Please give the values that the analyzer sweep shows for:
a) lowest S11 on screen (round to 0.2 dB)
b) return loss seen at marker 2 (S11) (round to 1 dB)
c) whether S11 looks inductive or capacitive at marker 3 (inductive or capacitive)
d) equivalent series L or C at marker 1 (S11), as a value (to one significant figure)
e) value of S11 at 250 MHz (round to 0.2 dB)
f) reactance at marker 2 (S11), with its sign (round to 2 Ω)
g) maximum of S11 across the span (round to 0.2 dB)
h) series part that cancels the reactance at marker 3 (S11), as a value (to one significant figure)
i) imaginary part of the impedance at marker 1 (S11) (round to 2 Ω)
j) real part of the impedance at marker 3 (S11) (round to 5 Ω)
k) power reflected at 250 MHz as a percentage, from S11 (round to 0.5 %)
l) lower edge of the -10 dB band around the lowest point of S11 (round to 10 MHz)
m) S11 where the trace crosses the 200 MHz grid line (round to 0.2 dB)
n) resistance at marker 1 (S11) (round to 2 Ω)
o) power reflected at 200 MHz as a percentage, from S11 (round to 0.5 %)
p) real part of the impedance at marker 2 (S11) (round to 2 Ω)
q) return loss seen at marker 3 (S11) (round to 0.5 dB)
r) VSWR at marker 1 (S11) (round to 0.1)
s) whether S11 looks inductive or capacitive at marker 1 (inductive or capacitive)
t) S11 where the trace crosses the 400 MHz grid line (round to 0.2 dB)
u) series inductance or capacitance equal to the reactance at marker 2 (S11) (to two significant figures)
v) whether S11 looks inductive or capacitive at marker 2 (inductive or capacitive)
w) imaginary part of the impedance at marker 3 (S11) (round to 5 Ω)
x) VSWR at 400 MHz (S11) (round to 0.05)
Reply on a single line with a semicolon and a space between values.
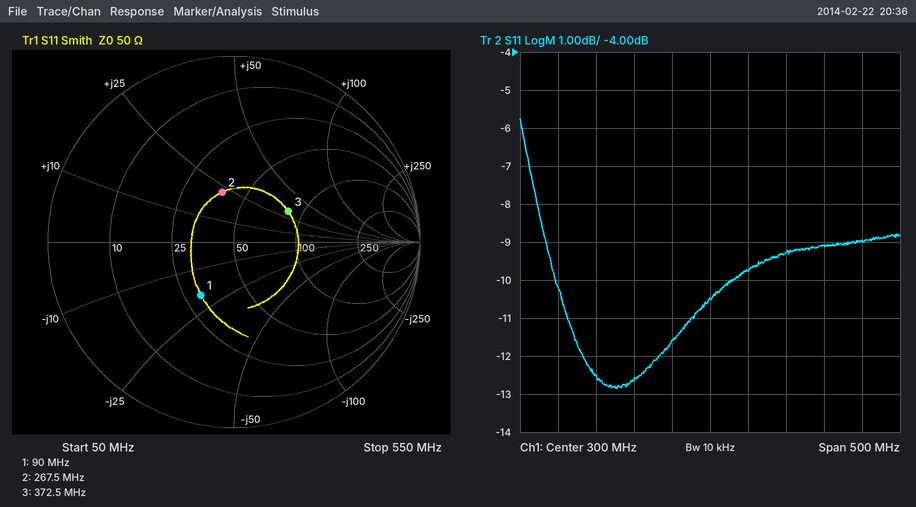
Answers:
-12.8 dB; 11 dB; inductive; 90 pF; -11.6 dB; +22 Ω; -5.8 dB; 10 pF; -20 Ω; 85 Ω; 7.0 %; 100 MHz; -12.6 dB; 30 Ω; 5.5 %; 38 Ω; 9.5 dB; 2.0; capacitive; -9.2 dB; 13 nH; inductive; +30 Ω; 2.05
